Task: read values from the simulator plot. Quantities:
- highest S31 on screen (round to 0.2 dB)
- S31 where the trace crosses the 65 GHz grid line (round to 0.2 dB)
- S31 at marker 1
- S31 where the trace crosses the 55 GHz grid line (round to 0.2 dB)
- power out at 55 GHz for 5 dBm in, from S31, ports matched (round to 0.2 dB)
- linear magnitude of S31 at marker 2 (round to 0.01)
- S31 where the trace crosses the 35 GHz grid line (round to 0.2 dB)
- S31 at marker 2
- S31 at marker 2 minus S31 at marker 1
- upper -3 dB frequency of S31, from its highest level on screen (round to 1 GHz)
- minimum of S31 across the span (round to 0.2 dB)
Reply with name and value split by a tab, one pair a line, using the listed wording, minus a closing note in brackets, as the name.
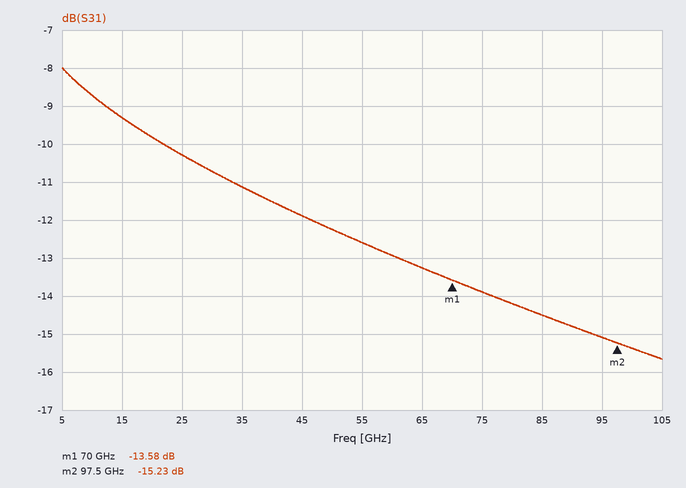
highest S31 on screen	-8.0 dB
S31 where the trace crosses the 65 GHz grid line	-13.2 dB
S31 at marker 1	-13.58 dB
S31 where the trace crosses the 55 GHz grid line	-12.6 dB
power out at 55 GHz for 5 dBm in, from S31, ports matched	-7.6 dBm
linear magnitude of S31 at marker 2	0.17
S31 where the trace crosses the 35 GHz grid line	-11.2 dB
S31 at marker 2	-15.23 dB
S31 at marker 2 minus S31 at marker 1	-1.65 dB
upper -3 dB frequency of S31, from its highest level on screen	33 GHz
minimum of S31 across the span	-15.6 dB
